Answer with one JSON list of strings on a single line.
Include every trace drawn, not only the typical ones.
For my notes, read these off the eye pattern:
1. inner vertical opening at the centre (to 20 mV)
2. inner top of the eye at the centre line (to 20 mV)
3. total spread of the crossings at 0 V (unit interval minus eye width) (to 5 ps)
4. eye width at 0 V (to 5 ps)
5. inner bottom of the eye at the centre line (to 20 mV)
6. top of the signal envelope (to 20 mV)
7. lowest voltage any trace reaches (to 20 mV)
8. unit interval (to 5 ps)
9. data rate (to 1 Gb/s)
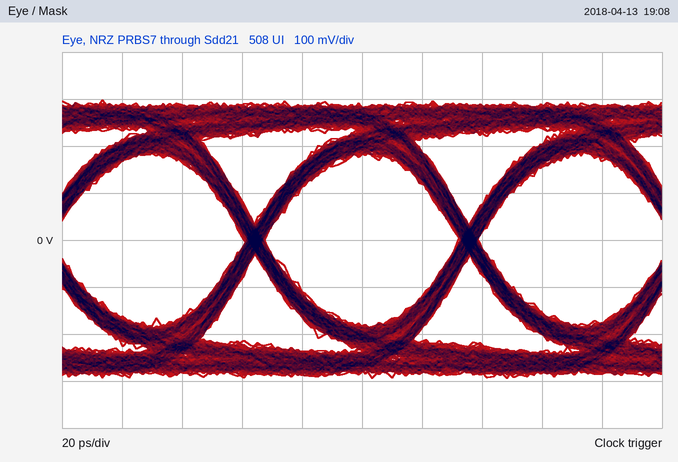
["360 mV", "180 mV", "5 ps", "65 ps", "-180 mV", "300 mV", "-300 mV", "70 ps", "14 Gb/s"]
